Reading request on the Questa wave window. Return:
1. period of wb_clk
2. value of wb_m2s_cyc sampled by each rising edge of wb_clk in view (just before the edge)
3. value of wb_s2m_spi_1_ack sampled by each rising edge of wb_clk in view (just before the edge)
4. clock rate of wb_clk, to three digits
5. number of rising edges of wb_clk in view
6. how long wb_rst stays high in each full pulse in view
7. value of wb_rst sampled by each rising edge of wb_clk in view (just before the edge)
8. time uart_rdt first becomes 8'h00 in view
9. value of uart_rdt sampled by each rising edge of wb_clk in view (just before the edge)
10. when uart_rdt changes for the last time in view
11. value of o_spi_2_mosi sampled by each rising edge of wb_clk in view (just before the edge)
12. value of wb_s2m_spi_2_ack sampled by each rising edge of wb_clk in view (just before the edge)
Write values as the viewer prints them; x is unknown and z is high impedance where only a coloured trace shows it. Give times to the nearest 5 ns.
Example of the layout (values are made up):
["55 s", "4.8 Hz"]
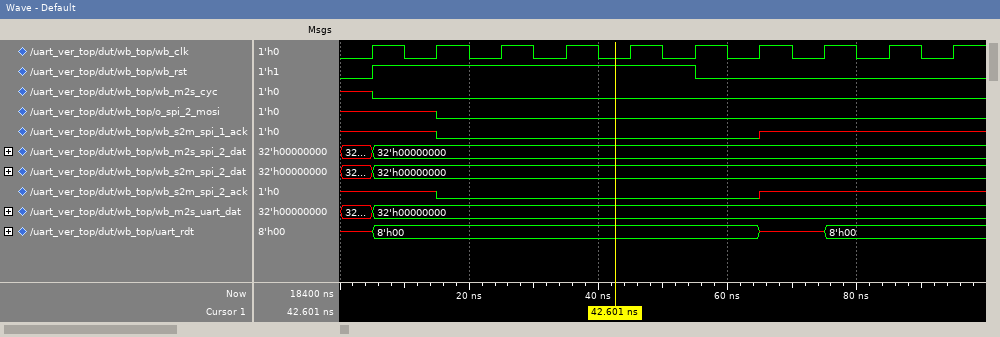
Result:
["10 ns", "x 0 0 0 0 0 0 0 0 0", "x x 0 0 0 0 0 x x x", "100 MHz", "10", "50 ns", "0 1 1 1 1 1 0 0 0 0", "5 ns", "x, 8'h00, 8'h00, 8'h00, 8'h00, 8'h00, 8'h00, x, 8'h00, 8'h00", "75 ns", "x x 0 0 0 0 0 0 0 0", "x x 0 0 0 0 0 x x x"]
